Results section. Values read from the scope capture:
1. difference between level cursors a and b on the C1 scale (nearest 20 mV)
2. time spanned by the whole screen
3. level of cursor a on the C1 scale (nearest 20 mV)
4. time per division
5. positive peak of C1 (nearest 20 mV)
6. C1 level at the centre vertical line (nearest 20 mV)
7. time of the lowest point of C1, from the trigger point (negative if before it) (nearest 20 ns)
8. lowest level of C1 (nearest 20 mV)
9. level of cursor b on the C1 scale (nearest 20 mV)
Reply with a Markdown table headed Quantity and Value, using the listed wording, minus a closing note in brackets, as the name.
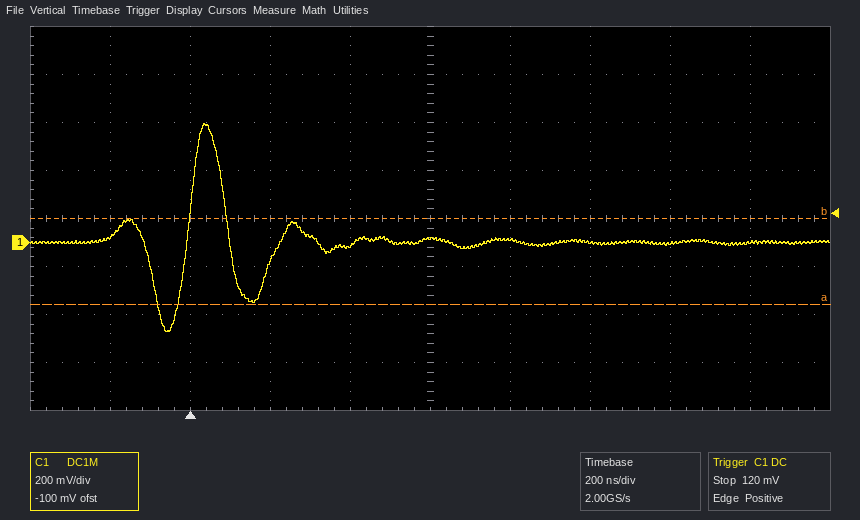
| Quantity | Value |
|---|---|
| difference between level cursors a and b on the C1 scale | 360 mV |
| time spanned by the whole screen | 2 µs |
| level of cursor a on the C1 scale | -260 mV |
| time per division | 200 ns |
| positive peak of C1 | 500 mV |
| C1 level at the centre vertical line | 20 mV |
| time of the lowest point of C1, from the trigger point (negative if before it) | -60 ns |
| lowest level of C1 | -380 mV |
| level of cursor b on the C1 scale | 100 mV |
